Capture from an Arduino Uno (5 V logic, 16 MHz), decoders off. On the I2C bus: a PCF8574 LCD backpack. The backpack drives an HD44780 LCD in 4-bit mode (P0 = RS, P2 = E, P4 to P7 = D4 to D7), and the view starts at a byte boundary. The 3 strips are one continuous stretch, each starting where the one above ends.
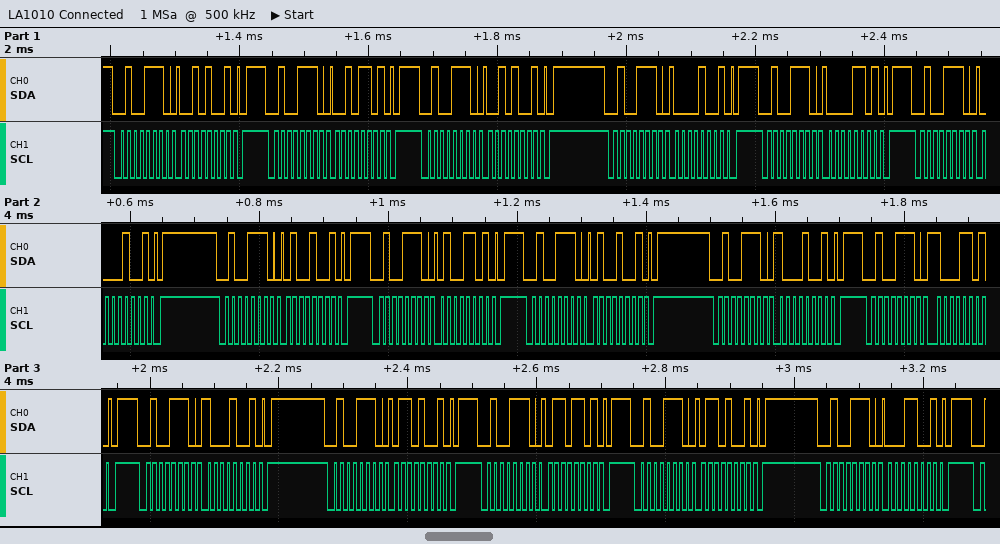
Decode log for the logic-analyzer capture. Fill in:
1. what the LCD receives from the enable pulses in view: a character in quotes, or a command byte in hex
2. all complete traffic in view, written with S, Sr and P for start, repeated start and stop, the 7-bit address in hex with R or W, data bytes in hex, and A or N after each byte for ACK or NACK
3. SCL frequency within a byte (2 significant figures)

' ' 'H'
S 27W A 29 A P S 27W A 2D A P S 27W A 29 A P S 27W A 09 A P S 27W A 0D A P S 27W A 09 A P S 27W A 49 A P S 27W A 4D A P S 27W A 49 A P S 27W A 89 A P S 27W A 8D A P S 27W A 89 A P S 27W A 69 A P S 27W A 6D A P S 27W A 69 A P S 27W A 19 A P
100 kHz
